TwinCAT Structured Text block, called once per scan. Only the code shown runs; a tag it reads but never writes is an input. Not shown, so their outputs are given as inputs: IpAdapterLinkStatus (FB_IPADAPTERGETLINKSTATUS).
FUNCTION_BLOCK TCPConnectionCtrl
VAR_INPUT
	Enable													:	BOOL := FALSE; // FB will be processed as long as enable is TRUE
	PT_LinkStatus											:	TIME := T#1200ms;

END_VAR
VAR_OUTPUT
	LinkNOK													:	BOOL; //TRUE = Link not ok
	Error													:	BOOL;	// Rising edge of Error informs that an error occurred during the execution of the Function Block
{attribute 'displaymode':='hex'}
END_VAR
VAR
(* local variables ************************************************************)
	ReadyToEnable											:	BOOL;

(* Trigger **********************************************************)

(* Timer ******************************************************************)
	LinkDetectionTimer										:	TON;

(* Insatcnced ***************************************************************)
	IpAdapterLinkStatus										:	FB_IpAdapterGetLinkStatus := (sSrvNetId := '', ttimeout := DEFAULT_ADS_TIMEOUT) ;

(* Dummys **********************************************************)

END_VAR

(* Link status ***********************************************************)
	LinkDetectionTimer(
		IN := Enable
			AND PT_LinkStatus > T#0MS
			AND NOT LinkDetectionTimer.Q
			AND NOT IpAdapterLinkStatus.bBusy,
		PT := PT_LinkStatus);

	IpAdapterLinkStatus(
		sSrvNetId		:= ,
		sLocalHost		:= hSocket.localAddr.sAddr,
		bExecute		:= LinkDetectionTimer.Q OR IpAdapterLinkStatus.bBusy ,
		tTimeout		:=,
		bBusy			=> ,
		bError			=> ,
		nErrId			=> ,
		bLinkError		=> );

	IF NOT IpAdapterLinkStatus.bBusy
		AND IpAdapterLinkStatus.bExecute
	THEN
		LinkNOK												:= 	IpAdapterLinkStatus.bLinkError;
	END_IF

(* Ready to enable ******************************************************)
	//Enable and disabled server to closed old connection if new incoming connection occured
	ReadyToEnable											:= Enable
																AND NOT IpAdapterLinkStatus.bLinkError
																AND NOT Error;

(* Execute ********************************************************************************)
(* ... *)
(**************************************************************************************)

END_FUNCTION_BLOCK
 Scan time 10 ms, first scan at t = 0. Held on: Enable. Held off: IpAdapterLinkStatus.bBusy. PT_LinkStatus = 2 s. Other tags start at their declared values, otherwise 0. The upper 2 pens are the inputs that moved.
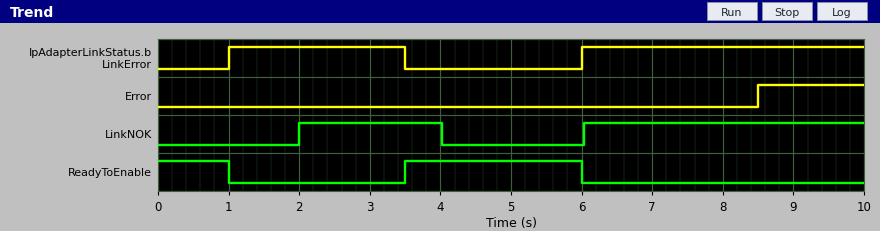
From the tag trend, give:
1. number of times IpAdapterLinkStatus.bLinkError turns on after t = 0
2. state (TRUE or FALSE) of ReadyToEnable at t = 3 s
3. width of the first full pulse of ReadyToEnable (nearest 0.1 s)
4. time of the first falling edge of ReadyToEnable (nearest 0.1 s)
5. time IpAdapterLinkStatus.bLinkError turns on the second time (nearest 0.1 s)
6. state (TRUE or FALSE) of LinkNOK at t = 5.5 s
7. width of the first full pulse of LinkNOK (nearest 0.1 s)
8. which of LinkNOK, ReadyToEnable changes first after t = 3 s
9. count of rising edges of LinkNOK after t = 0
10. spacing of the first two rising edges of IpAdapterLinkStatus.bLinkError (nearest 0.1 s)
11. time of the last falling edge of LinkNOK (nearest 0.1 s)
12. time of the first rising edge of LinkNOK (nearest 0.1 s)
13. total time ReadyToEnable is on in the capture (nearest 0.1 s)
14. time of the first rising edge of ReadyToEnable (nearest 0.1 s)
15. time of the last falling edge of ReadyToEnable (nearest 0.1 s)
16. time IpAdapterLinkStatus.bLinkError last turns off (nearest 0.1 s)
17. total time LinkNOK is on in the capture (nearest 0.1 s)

2
FALSE
2.5 s
1.0 s
6.0 s
FALSE
2.0 s
ReadyToEnable
2
5.0 s
4.0 s
2.0 s
3.5 s
3.5 s
6.0 s
3.5 s
6.0 s
